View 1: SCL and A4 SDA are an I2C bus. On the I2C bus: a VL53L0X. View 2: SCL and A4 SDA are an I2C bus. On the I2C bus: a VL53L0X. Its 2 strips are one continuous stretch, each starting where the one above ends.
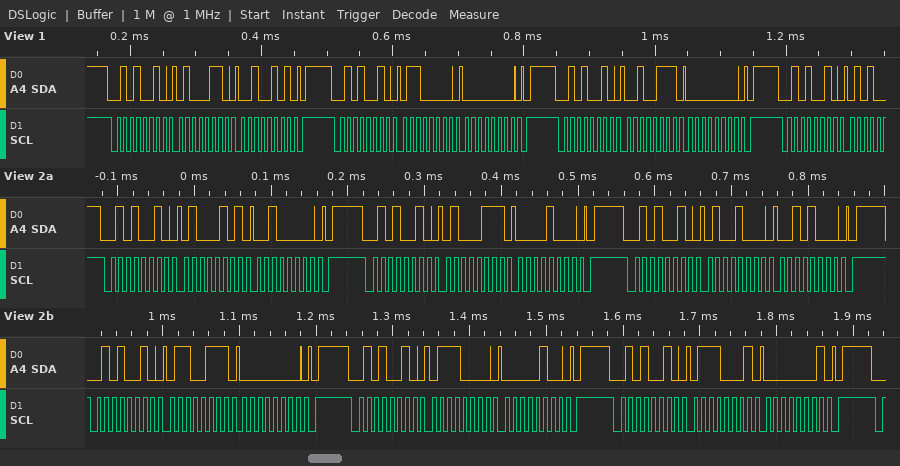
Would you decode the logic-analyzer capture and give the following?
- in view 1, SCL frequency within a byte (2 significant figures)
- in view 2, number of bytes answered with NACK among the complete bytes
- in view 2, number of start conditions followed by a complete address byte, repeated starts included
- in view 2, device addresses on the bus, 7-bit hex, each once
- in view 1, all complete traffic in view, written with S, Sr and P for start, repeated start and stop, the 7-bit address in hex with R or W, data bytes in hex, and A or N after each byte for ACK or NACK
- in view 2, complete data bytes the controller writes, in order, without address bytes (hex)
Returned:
100 kHz
0
6
0x29
S 29W A 46 A 25 A P S 29W A 60 A 00 A P S 29W A 27 A 00 A P S 29W A
45 20 47 08 48 28 67 00 70 04 71 01
